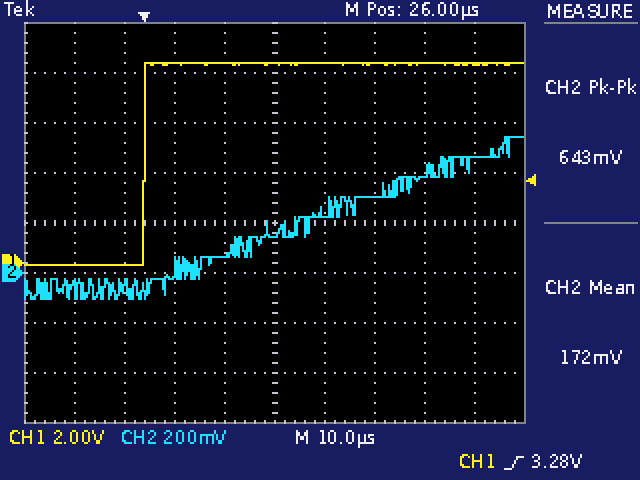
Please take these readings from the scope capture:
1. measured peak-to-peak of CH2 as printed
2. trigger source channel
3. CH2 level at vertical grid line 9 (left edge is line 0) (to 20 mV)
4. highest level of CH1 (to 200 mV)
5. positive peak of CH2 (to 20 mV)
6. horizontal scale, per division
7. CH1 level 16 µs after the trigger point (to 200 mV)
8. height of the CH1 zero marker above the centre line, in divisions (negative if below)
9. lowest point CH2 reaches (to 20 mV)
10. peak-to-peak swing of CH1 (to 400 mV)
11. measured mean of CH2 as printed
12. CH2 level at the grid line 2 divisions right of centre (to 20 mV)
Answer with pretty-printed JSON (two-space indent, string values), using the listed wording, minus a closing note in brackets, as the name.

{
  "measured peak-to-peak of CH2 as printed": "643 mV",
  "trigger source channel": "CH1",
  "CH2 level at vertical grid line 9 (left edge is line 0)": "460 mV",
  "highest level of CH1": "8.0 V",
  "positive peak of CH2": "540 mV",
  "horizontal scale, per division": "10 µs",
  "CH1 level 16 µs after the trigger point": "8.0 V",
  "height of the CH1 zero marker above the centre line, in divisions": "-0.8 div",
  "lowest point CH2 reaches": "-100 mV",
  "peak-to-peak swing of CH1": "8.0 V",
  "measured mean of CH2 as printed": "172 mV",
  "CH2 level at the grid line 2 divisions right of centre": "300 mV"
}
